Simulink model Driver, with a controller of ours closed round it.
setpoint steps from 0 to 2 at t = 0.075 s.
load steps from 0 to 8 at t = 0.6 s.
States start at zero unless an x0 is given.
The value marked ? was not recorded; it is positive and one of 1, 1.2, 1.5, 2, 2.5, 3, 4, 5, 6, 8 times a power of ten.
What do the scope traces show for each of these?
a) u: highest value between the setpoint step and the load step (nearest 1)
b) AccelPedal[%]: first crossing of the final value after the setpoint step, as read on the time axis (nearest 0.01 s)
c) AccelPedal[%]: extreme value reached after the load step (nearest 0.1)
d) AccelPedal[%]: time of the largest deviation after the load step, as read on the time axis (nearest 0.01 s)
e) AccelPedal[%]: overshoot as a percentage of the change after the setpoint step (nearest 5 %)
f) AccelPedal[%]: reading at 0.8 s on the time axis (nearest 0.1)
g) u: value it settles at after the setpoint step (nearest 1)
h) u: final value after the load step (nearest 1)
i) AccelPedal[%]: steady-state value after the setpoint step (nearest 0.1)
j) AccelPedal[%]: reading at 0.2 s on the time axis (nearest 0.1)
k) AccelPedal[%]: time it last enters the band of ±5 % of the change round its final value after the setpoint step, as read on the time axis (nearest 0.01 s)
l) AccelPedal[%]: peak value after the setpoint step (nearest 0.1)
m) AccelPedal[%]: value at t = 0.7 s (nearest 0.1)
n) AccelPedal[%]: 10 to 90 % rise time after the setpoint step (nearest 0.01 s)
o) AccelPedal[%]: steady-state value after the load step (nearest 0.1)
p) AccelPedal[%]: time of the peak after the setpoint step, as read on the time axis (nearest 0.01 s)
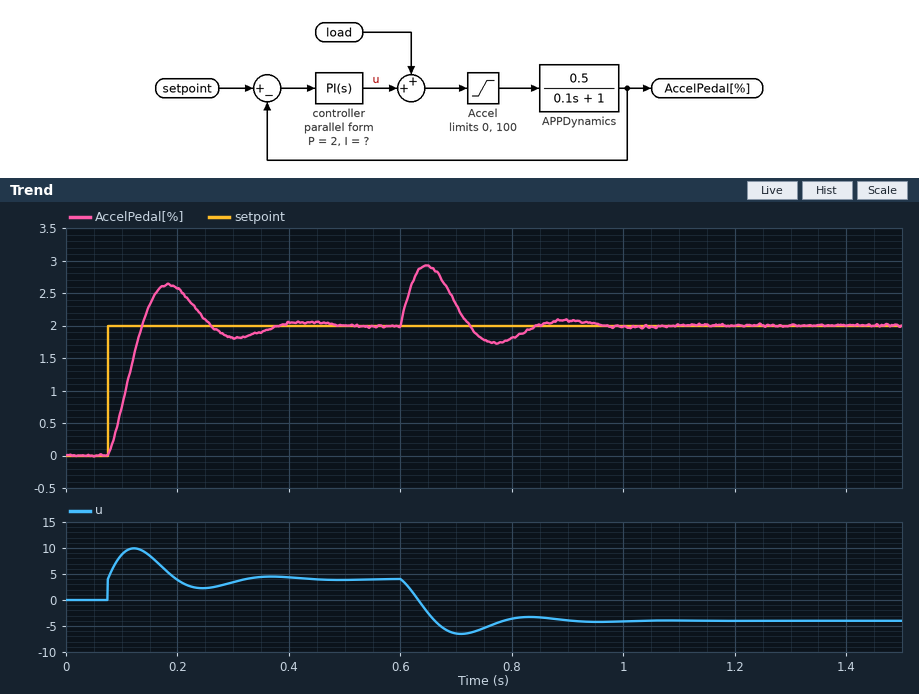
10
0.14 s
2.9
0.65 s
30 %
1.8
4
-4
2.0
2.6
0.35 s
2.6
2.3
0.05 s
2.0
0.18 s
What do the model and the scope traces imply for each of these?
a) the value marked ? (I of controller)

150
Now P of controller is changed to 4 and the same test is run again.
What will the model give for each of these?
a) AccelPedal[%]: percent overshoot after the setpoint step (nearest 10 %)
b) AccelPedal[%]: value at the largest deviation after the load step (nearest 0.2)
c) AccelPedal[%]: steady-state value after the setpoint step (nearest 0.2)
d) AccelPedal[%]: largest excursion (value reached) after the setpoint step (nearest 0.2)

20 %
2.8
2.0
2.4
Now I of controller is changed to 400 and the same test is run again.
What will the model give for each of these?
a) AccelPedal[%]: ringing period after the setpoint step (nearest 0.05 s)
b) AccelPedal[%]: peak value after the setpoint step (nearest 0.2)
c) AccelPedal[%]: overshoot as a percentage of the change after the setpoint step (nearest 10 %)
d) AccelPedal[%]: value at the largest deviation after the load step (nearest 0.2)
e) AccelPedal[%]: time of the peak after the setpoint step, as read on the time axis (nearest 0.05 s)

0.15 s
3.0
50 %
2.6
0.15 s
